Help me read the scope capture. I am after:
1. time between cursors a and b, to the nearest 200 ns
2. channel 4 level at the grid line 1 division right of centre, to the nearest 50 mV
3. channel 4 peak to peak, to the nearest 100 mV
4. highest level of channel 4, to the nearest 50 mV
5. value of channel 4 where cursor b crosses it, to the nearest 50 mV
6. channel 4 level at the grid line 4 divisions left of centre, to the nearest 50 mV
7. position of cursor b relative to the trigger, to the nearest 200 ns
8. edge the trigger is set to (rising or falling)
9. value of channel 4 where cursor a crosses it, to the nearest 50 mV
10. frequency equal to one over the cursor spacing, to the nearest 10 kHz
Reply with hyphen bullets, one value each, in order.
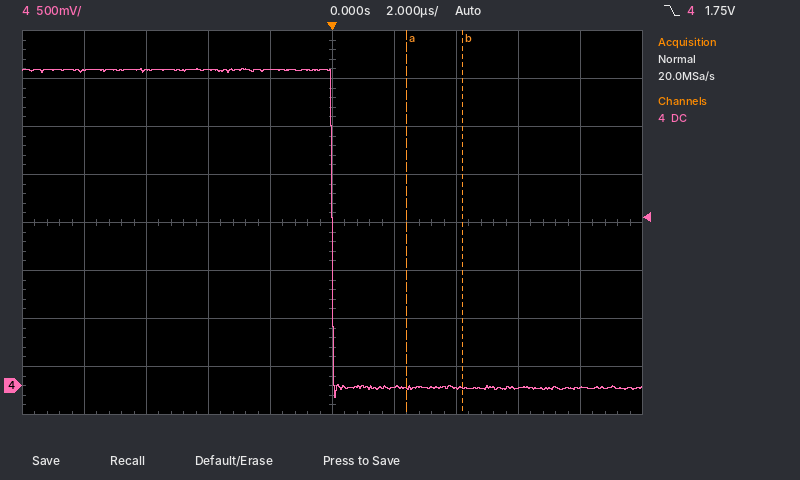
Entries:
- 1.8 µs
- 0 mV
- 3.40 V
- 3.30 V
- 0 mV
- 3.30 V
- +4.2 µs
- falling
- 0 mV
- 560 kHz
